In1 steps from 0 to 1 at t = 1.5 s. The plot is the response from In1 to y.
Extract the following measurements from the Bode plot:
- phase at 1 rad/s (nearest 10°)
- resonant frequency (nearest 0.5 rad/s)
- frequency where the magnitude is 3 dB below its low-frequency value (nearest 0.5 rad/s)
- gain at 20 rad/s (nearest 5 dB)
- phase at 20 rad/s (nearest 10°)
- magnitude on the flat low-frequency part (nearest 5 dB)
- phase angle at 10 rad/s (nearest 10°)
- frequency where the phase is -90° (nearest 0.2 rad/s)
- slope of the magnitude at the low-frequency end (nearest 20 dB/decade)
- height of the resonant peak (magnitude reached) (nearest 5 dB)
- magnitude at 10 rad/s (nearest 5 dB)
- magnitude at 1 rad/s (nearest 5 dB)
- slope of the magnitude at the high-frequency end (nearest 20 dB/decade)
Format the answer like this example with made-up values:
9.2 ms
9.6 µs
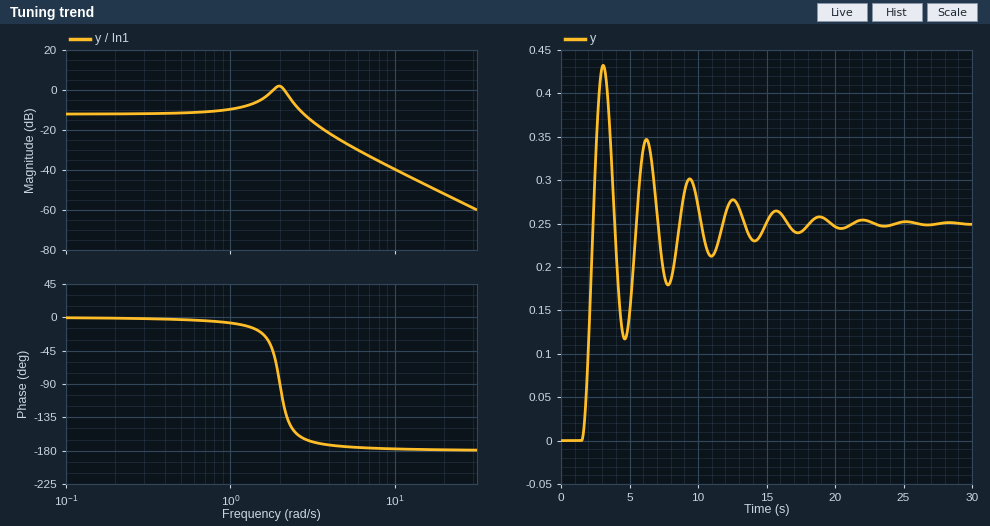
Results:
-10°
2.0 rad/s
3.0 rad/s
-50 dB
-180°
-10 dB
-180°
2.0 rad/s
0 dB/decade
0 dB
-40 dB
-10 dB
-40 dB/decade
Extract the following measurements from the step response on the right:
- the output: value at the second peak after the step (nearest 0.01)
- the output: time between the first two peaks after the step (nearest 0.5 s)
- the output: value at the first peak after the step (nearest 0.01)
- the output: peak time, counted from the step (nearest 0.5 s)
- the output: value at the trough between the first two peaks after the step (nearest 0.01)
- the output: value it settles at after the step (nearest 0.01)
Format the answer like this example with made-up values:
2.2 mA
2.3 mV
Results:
0.35
3.0 s
0.43
1.5 s
0.12
0.25
